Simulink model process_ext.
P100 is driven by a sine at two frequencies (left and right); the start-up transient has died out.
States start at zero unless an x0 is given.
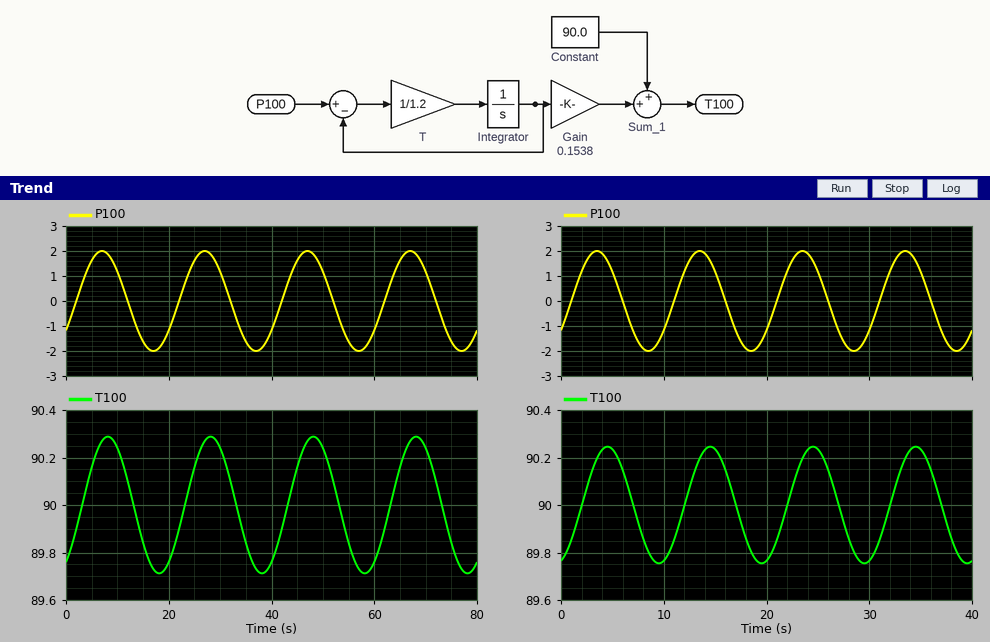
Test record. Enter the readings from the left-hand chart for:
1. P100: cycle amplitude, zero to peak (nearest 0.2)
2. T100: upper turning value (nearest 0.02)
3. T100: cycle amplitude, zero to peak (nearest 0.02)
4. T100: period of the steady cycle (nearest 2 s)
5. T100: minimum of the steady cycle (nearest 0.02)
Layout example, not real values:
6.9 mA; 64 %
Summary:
2.0; 90.28; 0.28; 20 s; 89.72
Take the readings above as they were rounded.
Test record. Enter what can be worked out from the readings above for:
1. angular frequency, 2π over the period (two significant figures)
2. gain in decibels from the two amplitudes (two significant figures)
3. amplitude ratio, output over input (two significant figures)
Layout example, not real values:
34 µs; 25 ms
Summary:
0.31 rad/s; -17 dB; 0.14
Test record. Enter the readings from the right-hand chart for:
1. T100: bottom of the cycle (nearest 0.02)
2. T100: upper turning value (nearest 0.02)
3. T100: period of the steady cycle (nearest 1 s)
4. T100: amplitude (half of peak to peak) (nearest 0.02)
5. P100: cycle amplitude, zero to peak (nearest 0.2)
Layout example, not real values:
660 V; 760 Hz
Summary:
89.76; 90.24; 10 s; 0.24; 2.0
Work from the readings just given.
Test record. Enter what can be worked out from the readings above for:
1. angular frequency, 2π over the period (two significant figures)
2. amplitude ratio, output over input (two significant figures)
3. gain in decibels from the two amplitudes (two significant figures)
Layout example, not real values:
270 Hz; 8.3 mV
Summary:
0.63 rad/s; 0.12; -18 dB
